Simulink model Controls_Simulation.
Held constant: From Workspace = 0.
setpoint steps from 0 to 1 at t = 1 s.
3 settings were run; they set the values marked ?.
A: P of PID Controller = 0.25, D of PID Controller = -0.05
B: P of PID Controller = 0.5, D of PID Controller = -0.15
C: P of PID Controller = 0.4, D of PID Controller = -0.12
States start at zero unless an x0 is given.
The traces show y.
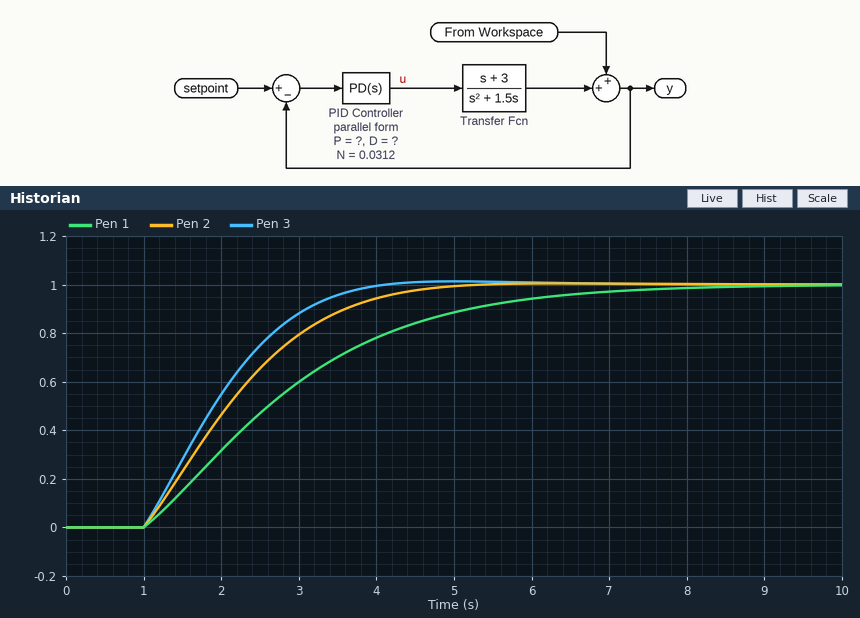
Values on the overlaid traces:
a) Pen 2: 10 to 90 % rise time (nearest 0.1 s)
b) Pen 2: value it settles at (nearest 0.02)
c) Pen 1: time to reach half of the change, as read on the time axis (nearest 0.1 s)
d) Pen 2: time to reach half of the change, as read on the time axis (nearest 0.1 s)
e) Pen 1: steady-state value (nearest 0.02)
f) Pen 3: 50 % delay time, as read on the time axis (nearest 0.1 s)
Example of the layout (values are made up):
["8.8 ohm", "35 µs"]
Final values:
["2.4 s", "1.00", "2.6 s", "2.1 s", "1.00", "1.9 s"]
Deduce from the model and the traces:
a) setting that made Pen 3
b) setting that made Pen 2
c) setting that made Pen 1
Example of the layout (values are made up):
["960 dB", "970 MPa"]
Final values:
["B", "C", "A"]
